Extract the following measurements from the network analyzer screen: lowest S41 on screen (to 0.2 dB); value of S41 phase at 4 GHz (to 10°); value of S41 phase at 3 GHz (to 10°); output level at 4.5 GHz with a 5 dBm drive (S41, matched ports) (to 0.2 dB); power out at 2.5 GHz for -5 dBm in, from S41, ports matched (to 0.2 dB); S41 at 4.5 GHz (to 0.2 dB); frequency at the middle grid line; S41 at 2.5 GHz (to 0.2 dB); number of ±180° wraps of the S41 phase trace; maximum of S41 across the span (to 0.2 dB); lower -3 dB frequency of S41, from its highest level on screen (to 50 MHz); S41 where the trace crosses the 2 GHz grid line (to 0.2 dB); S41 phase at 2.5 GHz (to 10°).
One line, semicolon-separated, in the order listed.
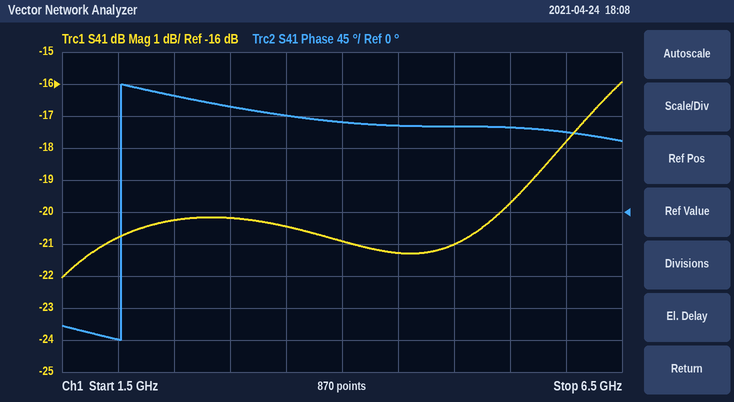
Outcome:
-22.0 dB; 130°; 150°; -16.2 dBm; -25.2 dBm; -21.2 dB; 4 GHz; -20.2 dB; 1; -16.0 dB; 5.70 GHz; -20.8 dB; 160°
